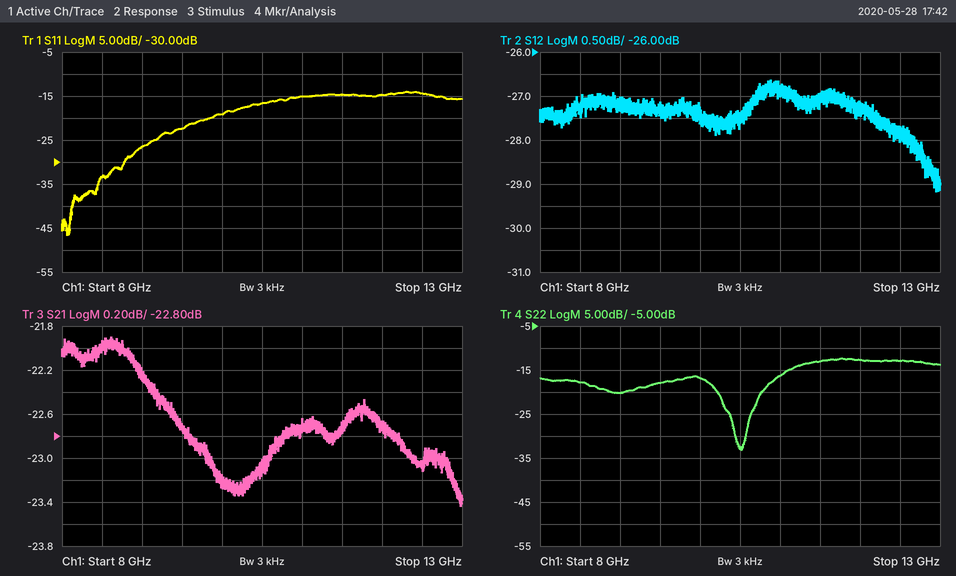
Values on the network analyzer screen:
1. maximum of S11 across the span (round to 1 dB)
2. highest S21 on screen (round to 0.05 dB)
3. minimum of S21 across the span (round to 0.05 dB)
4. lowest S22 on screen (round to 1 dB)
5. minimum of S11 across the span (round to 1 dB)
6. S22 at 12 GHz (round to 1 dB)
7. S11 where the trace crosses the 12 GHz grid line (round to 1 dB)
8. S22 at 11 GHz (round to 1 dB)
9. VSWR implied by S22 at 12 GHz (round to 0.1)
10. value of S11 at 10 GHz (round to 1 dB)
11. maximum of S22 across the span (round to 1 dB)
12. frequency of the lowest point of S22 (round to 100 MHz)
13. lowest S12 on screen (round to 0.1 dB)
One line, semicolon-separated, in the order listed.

-14 dB; -21.90 dB; -23.45 dB; -33 dB; -47 dB; -13 dB; -15 dB; -16 dB; 1.6; -19 dB; -12 dB; 10.5 GHz; -29.2 dB
